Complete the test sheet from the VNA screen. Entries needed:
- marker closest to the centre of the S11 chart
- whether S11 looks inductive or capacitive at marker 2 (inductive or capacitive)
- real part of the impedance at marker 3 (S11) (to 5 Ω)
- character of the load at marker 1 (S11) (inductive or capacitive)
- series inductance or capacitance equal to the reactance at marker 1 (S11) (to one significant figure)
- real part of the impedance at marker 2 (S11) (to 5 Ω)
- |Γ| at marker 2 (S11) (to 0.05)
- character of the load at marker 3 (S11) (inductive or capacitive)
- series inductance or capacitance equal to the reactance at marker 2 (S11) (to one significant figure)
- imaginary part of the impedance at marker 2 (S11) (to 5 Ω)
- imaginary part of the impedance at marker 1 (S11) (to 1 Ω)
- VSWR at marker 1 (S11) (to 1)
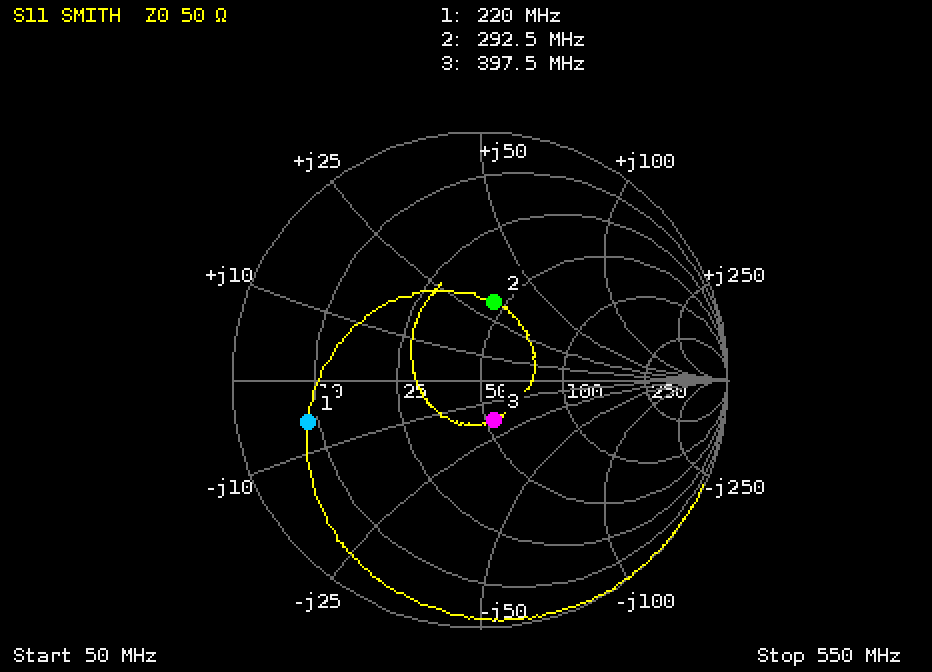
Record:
marker 3
inductive
55 Ω
capacitive
100 pF
45 Ω
0.30
capacitive
20 nH
+30 Ω
-6 Ω
6
